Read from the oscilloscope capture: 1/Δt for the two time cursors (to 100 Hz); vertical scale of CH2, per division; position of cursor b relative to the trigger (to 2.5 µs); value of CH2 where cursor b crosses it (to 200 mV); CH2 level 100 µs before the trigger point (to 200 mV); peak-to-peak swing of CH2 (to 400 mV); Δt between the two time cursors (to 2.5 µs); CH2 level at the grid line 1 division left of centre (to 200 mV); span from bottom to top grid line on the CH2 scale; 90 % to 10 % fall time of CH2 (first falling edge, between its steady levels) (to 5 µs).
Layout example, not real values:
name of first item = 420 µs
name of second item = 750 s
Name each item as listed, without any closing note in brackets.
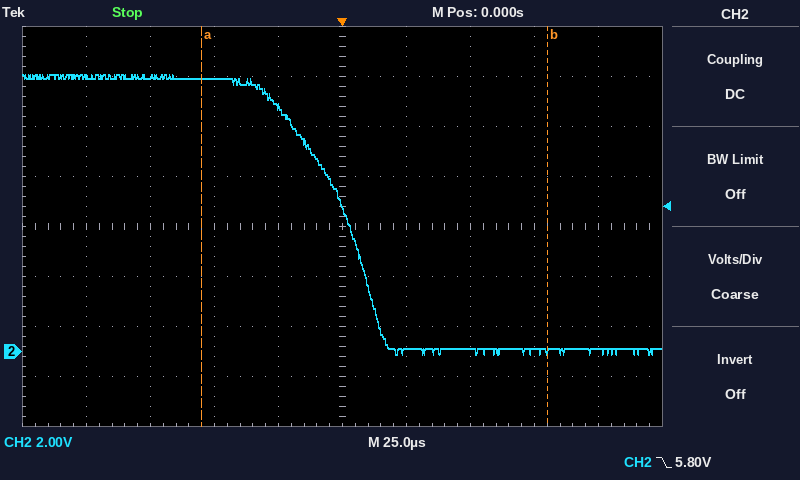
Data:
1/Δt for the two time cursors = 7.4 kHz
vertical scale of CH2, per division = 2 V
position of cursor b relative to the trigger = +80.0 µs
value of CH2 where cursor b crosses it = 0.0 V
CH2 level 100 µs before the trigger point = 11.0 V
peak-to-peak swing of CH2 = 11.2 V
Δt between the two time cursors = 135.0 µs
CH2 level at the grid line 1 division left of centre = 9.8 V
span from bottom to top grid line on the CH2 scale = 16 V
90 % to 10 % fall time of CH2 (first falling edge, between its steady levels) = 40 µs
